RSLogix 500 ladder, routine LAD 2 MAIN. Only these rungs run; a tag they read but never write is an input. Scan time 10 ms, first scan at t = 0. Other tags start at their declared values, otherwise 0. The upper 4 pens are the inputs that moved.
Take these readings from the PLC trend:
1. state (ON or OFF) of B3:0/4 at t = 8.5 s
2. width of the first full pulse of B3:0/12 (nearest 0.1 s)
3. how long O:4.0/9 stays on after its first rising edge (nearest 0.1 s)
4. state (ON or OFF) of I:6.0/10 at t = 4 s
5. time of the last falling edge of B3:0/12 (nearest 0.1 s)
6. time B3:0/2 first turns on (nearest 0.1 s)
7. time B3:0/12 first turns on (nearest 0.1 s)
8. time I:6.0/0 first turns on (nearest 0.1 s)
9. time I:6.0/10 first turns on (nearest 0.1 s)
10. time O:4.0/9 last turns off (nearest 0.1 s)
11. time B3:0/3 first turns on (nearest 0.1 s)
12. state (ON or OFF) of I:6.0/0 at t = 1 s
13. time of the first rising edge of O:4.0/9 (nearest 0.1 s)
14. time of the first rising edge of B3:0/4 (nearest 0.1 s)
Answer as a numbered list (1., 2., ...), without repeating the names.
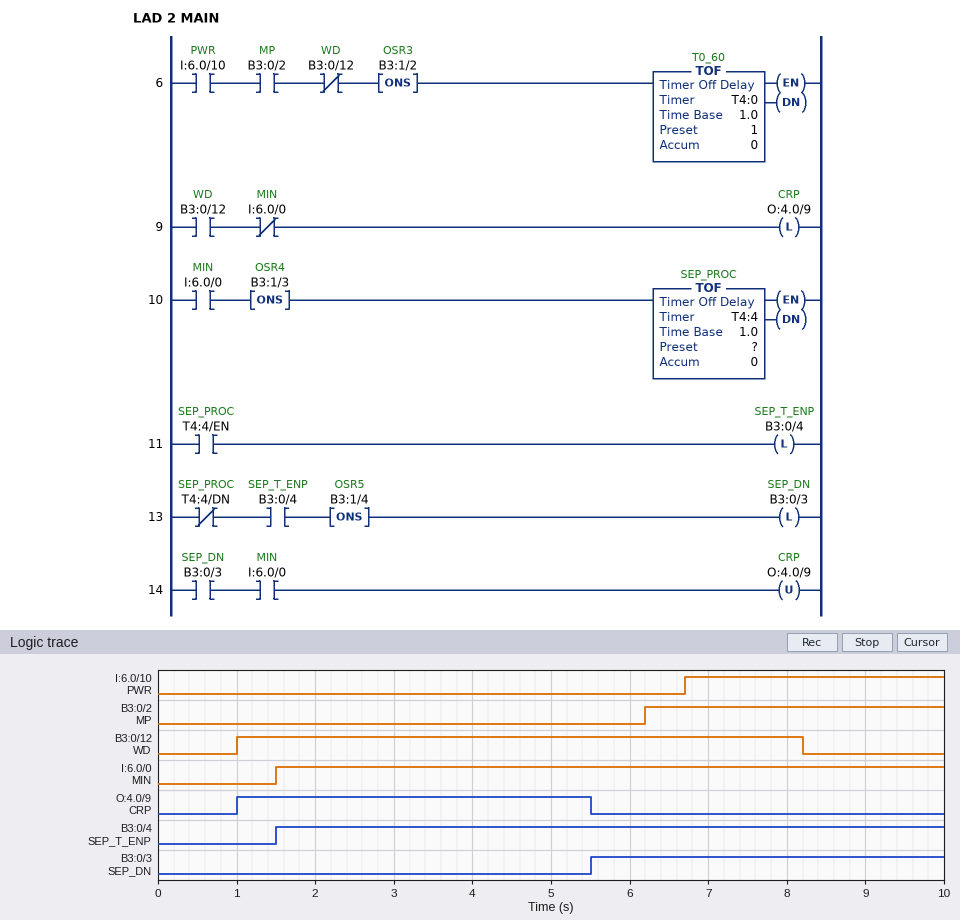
1. ON
2. 7.2 s
3. 4.5 s
4. OFF
5. 8.2 s
6. 6.2 s
7. 1.0 s
8. 1.5 s
9. 6.7 s
10. 5.5 s
11. 5.5 s
12. OFF
13. 1.0 s
14. 1.5 s
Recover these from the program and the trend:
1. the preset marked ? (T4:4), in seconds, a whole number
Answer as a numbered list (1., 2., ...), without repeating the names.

1. 4 s
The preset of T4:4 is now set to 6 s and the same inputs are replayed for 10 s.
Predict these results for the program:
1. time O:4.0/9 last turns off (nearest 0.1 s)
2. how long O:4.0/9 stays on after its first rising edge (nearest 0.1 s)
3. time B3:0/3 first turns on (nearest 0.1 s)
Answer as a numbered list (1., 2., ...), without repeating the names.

1. 7.5 s
2. 6.5 s
3. 7.5 s
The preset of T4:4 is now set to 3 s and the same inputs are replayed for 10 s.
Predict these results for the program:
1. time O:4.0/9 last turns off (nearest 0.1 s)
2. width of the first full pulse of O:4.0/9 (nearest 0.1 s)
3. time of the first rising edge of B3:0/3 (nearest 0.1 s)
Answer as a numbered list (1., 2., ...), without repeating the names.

1. 4.5 s
2. 3.5 s
3. 4.5 s
